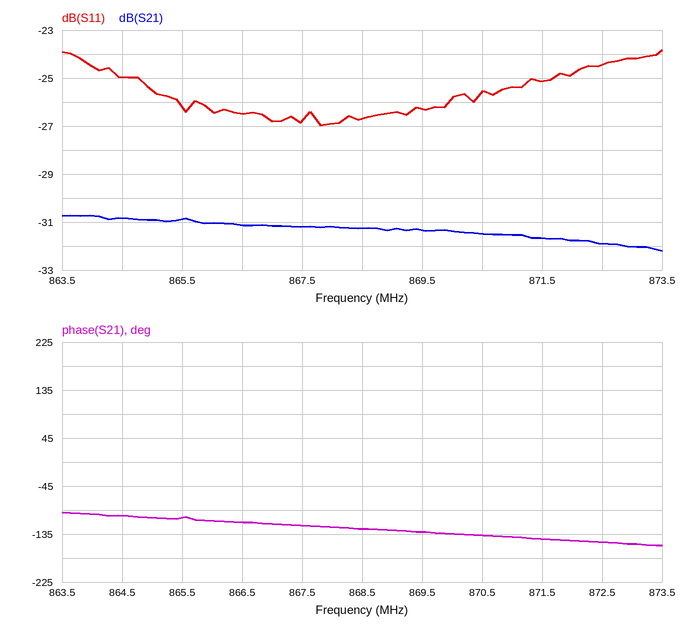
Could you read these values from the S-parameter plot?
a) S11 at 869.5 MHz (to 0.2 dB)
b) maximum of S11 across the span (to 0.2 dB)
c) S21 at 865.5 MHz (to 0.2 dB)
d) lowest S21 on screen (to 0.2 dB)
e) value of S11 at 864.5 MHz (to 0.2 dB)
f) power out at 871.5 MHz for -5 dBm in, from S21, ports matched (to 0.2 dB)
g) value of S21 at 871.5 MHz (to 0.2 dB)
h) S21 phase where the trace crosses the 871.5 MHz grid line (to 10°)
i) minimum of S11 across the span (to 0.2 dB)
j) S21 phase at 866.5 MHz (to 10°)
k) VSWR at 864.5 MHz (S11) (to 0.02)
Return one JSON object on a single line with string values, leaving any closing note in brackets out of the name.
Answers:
{"S11 at 869.5 MHz": "-26.2 dB", "maximum of S11 across the span": "-23.8 dB", "S21 at 865.5 MHz": "-30.8 dB", "lowest S21 on screen": "-32.2 dB", "value of S11 at 864.5 MHz": "-25.0 dB", "power out at 871.5 MHz for -5 dBm in, from S21, ports matched": "-36.6 dBm", "value of S21 at 871.5 MHz": "-31.6 dB", "S21 phase where the trace crosses the 871.5 MHz grid line": "-140°", "minimum of S11 across the span": "-27.0 dB", "S21 phase at 866.5 MHz": "-110°", "VSWR at 864.5 MHz (S11)": "1.12"}
